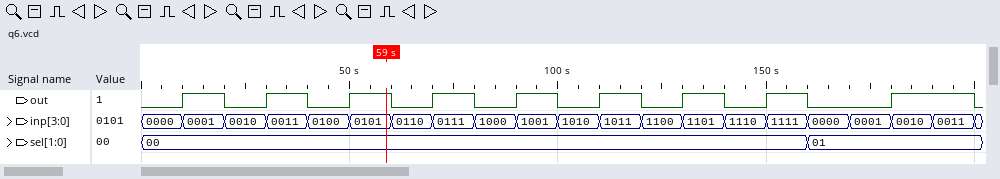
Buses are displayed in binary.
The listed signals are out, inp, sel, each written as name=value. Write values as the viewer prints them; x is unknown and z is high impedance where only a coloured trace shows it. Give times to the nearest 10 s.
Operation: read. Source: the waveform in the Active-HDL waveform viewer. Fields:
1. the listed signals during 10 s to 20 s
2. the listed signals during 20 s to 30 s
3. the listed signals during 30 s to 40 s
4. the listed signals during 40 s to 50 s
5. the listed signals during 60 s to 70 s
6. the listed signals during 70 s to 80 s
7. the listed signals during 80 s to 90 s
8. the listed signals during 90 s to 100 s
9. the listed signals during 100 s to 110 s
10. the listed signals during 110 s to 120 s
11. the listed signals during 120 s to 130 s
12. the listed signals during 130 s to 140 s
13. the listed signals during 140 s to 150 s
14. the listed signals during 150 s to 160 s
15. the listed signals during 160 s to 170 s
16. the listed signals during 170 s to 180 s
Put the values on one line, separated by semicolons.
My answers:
out=1, inp=0001, sel=00; out=0, inp=0010, sel=00; out=1, inp=0011, sel=00; out=0, inp=0100, sel=00; out=0, inp=0110, sel=00; out=1, inp=0111, sel=00; out=0, inp=1000, sel=00; out=1, inp=1001, sel=00; out=0, inp=1010, sel=00; out=1, inp=1011, sel=00; out=0, inp=1100, sel=00; out=1, inp=1101, sel=00; out=0, inp=1110, sel=00; out=1, inp=1111, sel=00; out=0, inp=0000, sel=01; out=0, inp=0001, sel=01
